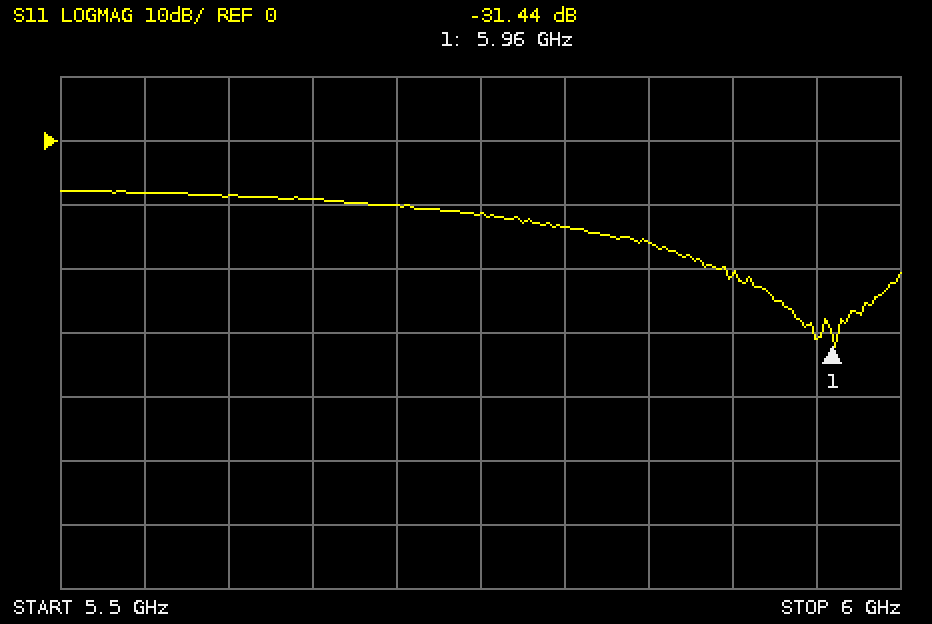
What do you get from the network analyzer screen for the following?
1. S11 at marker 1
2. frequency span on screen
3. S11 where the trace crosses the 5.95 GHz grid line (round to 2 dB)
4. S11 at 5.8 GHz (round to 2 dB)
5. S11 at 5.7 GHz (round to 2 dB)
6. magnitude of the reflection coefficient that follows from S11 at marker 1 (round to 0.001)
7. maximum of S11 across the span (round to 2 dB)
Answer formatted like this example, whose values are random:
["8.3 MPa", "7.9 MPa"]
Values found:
["-31.44 dB", "500 MHz", "-30 dB", "-14 dB", "-10 dB", "0.027", "-8 dB"]
